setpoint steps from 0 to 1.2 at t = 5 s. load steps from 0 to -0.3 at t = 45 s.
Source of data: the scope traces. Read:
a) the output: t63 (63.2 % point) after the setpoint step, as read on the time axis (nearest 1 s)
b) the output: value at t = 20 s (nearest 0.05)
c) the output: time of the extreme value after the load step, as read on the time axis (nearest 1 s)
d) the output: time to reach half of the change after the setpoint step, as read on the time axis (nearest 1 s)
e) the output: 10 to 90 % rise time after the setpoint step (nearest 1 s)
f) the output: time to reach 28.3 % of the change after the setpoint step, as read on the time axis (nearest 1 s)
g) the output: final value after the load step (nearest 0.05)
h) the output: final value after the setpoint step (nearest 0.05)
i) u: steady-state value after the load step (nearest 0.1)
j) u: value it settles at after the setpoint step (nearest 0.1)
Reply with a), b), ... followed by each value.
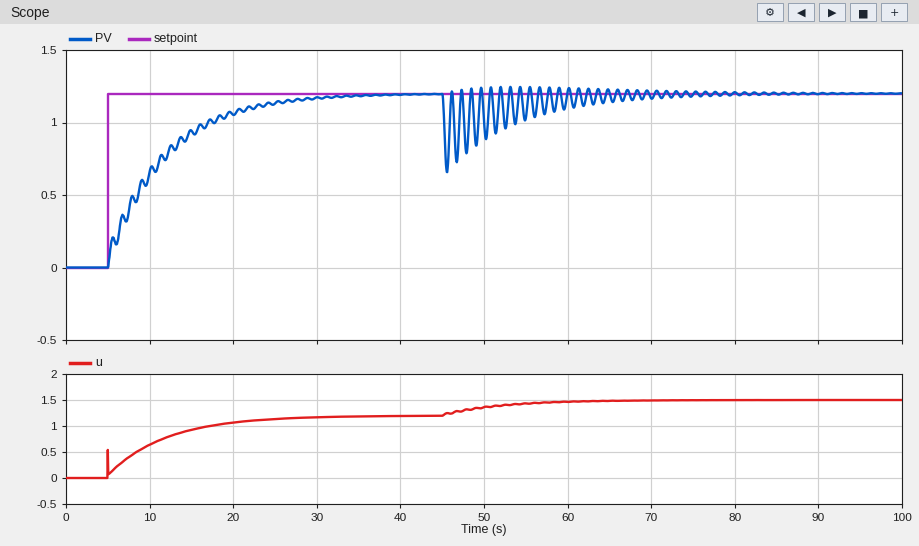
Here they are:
a) 11 s
b) 1.05
c) 46 s
d) 9 s
e) 15 s
f) 7 s
g) 1.20
h) 1.20
i) 1.5
j) 1.2
